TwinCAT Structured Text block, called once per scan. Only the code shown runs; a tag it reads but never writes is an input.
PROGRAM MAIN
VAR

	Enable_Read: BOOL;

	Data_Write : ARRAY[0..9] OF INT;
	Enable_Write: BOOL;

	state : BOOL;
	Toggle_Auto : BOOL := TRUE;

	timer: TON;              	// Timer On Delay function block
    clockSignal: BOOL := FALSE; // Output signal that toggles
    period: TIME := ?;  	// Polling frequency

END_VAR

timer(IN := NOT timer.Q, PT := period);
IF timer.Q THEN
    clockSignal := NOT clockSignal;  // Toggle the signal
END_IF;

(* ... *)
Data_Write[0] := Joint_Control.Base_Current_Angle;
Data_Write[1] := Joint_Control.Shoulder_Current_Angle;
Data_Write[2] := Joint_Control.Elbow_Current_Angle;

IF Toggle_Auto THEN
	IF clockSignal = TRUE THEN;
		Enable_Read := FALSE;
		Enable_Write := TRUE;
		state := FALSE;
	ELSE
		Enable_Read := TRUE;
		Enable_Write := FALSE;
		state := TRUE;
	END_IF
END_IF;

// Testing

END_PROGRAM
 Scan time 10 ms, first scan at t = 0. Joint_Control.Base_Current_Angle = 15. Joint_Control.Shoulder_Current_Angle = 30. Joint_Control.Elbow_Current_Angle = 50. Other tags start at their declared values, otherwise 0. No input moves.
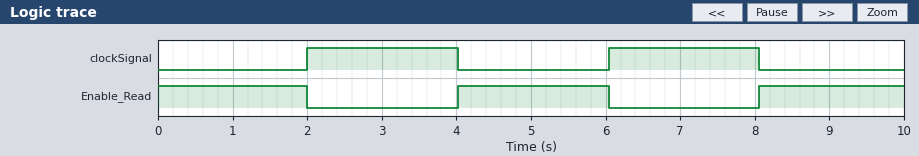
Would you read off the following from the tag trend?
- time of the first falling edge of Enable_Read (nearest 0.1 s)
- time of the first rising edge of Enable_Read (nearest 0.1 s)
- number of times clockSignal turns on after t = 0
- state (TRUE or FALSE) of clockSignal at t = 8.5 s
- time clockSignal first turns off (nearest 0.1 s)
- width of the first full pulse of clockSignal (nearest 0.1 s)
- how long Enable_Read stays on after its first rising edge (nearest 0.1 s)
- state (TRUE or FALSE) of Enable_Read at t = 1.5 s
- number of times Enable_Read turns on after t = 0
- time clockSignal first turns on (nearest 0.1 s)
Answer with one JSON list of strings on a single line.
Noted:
["2.0 s", "4.0 s", "2", "FALSE", "4.0 s", "2.0 s", "2.0 s", "TRUE", "2", "2.0 s"]
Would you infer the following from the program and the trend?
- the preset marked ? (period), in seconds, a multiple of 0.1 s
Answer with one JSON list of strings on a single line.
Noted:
["2.0 s"]
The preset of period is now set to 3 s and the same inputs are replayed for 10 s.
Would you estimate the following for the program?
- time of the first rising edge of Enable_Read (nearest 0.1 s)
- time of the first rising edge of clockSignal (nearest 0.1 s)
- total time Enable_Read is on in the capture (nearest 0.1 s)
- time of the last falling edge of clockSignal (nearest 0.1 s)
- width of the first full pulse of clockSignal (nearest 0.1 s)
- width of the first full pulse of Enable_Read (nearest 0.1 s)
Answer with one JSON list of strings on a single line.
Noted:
["6.0 s", "3.0 s", "6.0 s", "6.0 s", "3.0 s", "3.0 s"]
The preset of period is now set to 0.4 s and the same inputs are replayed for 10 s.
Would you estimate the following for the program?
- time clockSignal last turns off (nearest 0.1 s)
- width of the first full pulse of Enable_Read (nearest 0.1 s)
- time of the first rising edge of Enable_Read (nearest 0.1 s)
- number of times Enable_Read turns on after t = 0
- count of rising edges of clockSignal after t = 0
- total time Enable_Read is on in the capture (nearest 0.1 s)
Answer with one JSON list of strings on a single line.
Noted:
["9.2 s", "0.4 s", "0.8 s", "11", "12", "5.0 s"]
